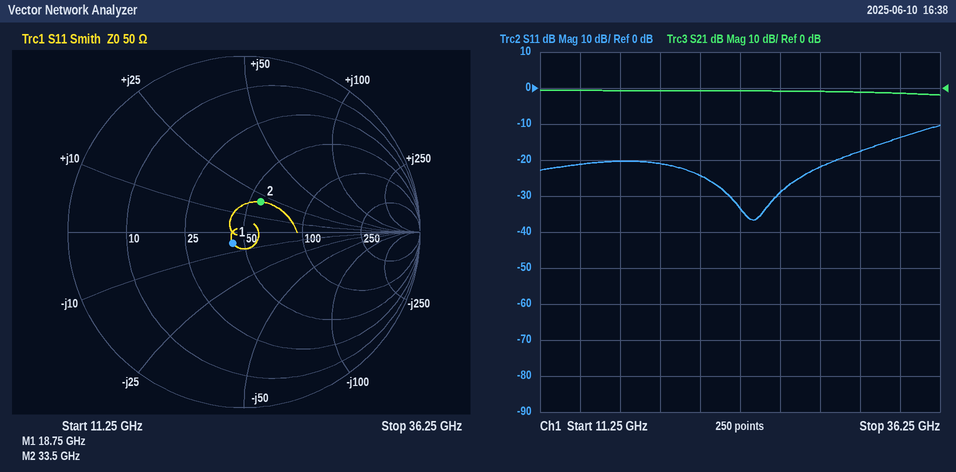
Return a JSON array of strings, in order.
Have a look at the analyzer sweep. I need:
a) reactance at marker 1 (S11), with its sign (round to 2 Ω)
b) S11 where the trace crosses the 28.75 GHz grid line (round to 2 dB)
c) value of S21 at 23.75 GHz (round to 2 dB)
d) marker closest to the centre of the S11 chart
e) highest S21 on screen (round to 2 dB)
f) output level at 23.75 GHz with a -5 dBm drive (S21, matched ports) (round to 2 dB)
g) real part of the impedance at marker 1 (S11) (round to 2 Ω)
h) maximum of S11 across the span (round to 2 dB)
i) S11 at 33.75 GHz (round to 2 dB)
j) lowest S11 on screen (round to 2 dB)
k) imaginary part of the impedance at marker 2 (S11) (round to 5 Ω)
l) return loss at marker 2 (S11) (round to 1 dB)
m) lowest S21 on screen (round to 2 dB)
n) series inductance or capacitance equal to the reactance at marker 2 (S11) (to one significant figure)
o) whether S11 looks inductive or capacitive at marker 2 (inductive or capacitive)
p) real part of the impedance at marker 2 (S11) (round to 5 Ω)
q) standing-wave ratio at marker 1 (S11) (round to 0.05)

["-6 Ω", "-22 dB", "0 dB", "marker 1", "0 dB", "-6 dBm", "44 Ω", "-10 dB", "-14 dB", "-36 dB", "+20 Ω", "14 dB", "-2 dB", "100 pH", "inductive", "55 Ω", "1.20"]
